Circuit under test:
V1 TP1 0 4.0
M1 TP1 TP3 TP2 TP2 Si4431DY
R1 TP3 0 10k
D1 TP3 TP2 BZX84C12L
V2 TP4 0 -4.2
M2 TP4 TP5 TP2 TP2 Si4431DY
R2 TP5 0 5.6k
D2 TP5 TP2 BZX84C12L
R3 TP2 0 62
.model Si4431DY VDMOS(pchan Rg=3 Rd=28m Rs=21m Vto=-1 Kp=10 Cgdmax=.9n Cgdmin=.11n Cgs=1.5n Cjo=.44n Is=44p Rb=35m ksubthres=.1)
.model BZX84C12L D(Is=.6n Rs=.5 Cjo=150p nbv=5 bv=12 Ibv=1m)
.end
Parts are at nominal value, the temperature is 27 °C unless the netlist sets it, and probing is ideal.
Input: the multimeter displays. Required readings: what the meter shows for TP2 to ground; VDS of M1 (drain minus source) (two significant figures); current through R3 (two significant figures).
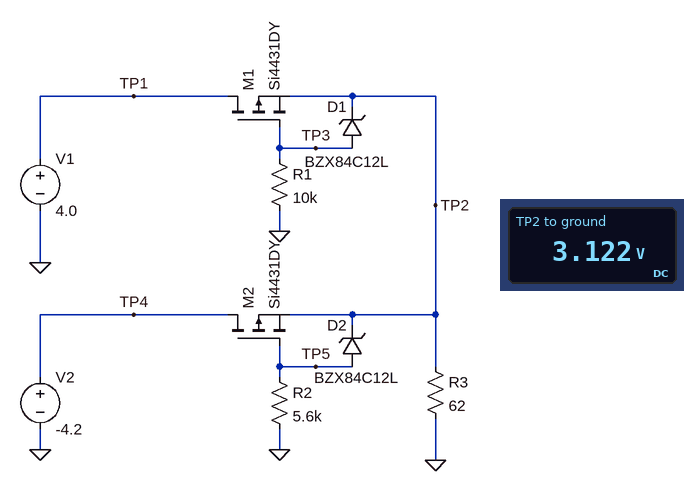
3.122 V
880 mV
50 mA
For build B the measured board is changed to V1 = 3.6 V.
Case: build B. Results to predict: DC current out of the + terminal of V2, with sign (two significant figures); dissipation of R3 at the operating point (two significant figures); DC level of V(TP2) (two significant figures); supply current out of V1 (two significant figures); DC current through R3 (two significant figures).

-12 A
130 mW
2.8 V
12 A
45 mA
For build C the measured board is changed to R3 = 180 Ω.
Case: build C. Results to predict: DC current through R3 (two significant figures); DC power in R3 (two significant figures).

17 mA
54 mW
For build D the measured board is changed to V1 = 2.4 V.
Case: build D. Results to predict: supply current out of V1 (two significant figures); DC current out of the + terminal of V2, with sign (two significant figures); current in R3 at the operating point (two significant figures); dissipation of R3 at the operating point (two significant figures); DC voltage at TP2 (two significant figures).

3.6 A
-3.5 A
31 mA
59 mW
1.9 V
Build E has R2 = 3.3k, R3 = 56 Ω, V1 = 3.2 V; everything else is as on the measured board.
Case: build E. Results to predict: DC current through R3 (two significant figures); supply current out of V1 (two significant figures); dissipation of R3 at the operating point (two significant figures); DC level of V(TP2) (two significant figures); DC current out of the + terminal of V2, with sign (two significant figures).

45 mA
8.7 A
110 mW
2.5 V
-8.7 A
